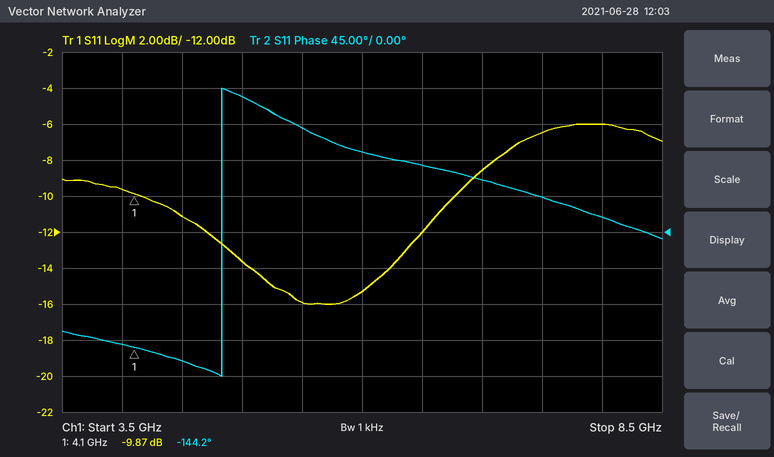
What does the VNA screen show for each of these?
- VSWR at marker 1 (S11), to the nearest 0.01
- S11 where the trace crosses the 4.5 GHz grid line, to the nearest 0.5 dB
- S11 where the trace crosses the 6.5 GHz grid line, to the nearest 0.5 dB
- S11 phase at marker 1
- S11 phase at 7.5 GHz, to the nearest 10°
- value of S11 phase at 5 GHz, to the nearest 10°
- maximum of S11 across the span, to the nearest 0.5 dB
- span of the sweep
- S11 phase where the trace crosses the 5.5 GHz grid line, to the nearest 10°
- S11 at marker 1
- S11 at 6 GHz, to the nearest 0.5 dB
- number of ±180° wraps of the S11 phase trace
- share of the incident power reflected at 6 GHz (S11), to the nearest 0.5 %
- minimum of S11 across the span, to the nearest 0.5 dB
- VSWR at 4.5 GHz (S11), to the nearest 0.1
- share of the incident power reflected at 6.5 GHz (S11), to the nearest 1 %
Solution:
1.95
-11.0 dB
-12.0 dB
-144.2°
40°
170°
-6.0 dB
5 GHz
130°
-9.87 dB
-15.5 dB
1
3.0 %
-16.0 dB
1.8
6 %
